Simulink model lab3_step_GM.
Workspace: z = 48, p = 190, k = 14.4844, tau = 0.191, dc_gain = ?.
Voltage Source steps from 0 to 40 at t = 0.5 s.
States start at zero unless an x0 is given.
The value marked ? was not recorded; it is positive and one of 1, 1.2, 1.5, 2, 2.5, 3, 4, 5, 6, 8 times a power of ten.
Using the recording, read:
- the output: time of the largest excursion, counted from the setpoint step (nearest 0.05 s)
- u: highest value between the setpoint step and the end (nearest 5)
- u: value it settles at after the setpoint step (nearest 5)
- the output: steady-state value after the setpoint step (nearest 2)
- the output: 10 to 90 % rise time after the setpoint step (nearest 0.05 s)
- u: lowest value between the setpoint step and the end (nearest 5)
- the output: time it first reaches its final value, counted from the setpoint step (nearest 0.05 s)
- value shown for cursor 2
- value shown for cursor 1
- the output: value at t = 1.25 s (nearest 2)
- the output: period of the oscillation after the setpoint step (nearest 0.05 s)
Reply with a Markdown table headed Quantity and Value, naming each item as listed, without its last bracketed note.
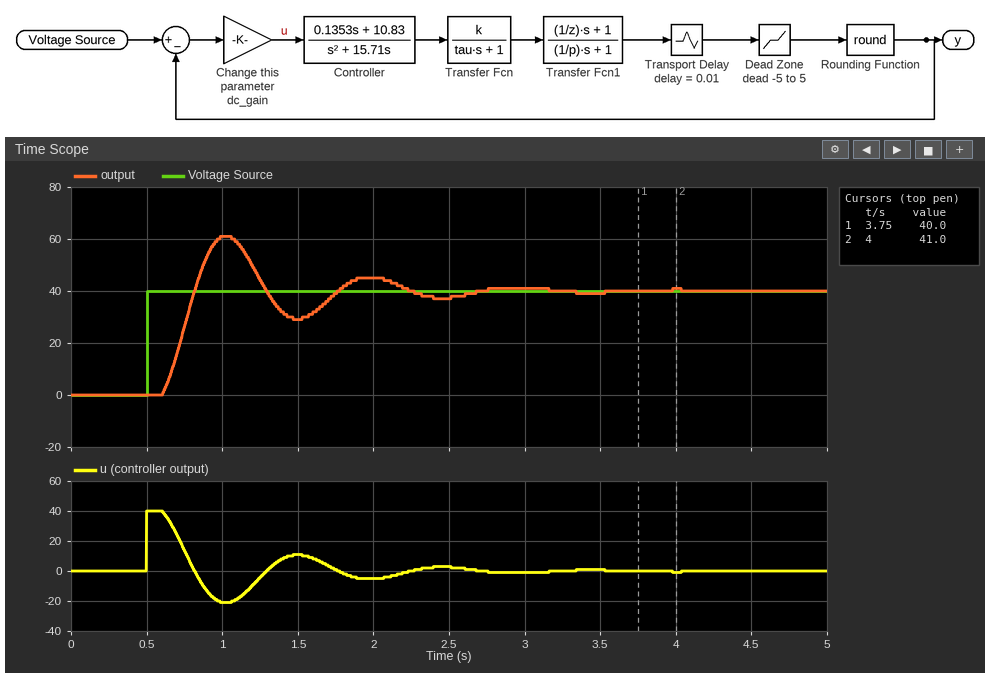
| Quantity | Value |
|---|---|
| the output: time of the largest excursion, counted from the setpoint step | 0.50 s |
| u: highest value between the setpoint step and the end | 40 |
| u: value it settles at after the setpoint step | 0 |
| the output: steady-state value after the setpoint step | 40 |
| the output: 10 to 90 % rise time after the setpoint step | 0.15 s |
| u: lowest value between the setpoint step and the end | -20 |
| the output: time it first reaches its final value, counted from the setpoint step | 0.30 s |
| value shown for cursor 2 | 41.0 |
| value shown for cursor 1 | 40.0 |
| the output: value at t = 1.25 s | 44 |
| the output: period of the oscillation after the setpoint step | 0.95 s |
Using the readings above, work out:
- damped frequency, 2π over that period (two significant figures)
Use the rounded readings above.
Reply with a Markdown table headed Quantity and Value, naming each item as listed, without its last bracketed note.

| Quantity | Value |
|---|---|
| damped frequency, 2π over that period | 6.6 rad/s |
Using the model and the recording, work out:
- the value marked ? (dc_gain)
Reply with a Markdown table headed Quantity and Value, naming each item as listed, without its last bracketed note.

| Quantity | Value |
|---|---|
| the value marked ? | 1 |
